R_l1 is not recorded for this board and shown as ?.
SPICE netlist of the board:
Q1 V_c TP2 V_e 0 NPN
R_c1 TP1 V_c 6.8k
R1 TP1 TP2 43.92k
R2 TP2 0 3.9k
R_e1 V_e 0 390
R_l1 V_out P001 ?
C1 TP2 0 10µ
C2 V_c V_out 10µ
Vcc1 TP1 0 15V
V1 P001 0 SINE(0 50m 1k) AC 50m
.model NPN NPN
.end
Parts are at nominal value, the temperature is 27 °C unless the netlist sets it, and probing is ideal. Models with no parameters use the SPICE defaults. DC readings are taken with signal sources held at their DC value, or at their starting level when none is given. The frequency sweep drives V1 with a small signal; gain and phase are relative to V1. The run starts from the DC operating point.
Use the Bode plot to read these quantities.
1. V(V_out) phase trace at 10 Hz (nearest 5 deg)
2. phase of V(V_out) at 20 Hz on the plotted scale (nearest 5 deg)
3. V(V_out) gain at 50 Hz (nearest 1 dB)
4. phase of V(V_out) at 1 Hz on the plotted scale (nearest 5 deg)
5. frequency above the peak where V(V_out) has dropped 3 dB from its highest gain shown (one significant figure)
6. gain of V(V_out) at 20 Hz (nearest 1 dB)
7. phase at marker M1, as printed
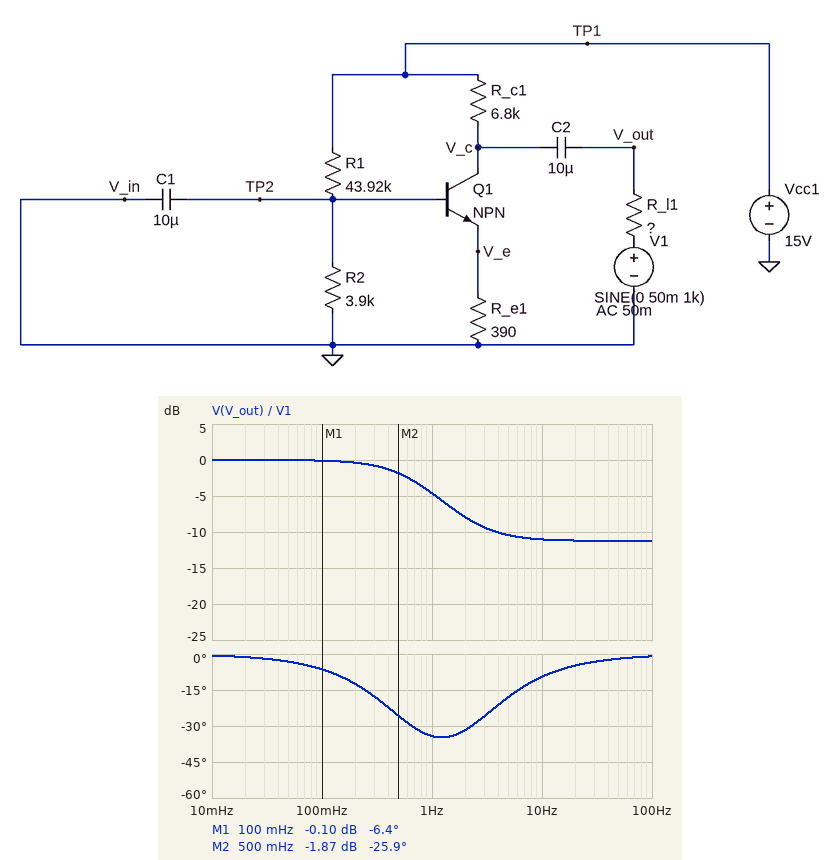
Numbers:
-10 deg
-5 deg
-11 dB
-35 deg
700 mHz
-11 dB
-6.4 deg
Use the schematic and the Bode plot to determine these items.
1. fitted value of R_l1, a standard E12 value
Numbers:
18 kΩ
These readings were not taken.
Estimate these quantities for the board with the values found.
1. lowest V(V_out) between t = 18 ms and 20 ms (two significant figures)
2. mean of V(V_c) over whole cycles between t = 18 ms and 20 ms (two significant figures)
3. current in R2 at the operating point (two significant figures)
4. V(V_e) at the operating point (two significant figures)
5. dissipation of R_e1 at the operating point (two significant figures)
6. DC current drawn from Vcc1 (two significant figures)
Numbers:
-14 mV
7.9 V
300 µA
410 mV
430 µW
1.4 mA
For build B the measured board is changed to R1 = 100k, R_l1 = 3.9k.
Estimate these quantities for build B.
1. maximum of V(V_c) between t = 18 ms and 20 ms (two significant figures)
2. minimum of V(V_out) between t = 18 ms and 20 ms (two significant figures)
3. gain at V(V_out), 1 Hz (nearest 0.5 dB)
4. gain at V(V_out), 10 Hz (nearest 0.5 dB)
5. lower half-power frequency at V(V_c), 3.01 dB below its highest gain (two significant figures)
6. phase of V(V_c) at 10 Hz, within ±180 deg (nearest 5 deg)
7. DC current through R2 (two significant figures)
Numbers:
15 V
-32 mV
-1.0 dB
-4.0 dB
1.5 Hz
10 deg
140 µA
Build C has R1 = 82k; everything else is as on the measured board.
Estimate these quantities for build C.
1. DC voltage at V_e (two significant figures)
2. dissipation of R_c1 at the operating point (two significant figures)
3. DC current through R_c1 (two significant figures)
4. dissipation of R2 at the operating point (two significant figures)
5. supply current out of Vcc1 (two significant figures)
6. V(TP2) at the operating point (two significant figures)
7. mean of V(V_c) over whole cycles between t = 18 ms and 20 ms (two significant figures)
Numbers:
7.7 mV
2.6 µW
20 µA
120 µW
190 µA
680 mV
15 V
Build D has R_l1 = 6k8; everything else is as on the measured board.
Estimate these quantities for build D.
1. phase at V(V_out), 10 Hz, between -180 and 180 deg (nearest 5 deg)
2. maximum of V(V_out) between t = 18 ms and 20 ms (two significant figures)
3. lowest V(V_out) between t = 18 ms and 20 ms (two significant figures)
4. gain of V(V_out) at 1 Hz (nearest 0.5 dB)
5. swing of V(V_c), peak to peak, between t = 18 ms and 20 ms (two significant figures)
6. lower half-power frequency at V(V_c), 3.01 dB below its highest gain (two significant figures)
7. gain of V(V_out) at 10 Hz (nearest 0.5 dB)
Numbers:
-5 deg
25 mV
-25 mV
-1.5 dB
50 mV
1.2 Hz
-6.0 dB
